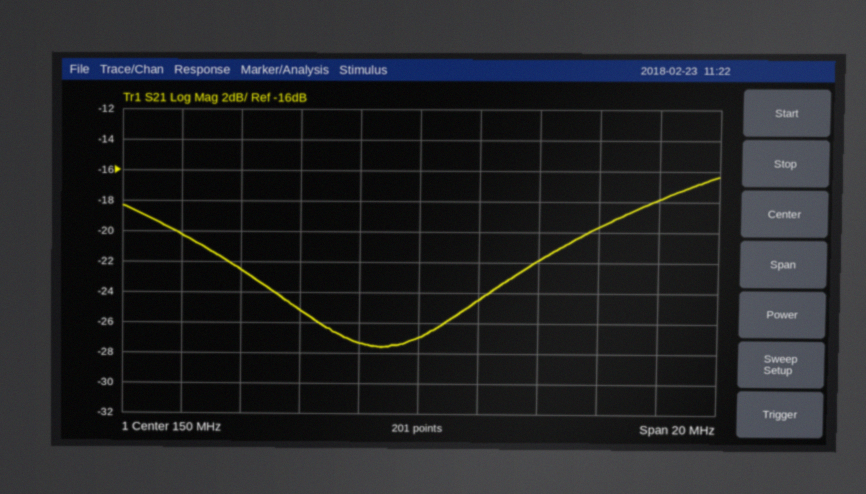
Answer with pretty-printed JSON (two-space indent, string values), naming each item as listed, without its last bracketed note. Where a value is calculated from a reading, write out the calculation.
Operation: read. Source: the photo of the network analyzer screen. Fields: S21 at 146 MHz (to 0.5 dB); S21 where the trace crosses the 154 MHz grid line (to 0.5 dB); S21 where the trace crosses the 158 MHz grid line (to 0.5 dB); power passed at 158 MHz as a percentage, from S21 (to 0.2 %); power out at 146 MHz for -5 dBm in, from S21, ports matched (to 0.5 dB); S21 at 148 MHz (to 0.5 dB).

{
  "S21 at 146 MHz": "-25.0 dB",
  "S21 where the trace crosses the 154 MHz grid line": "-22.0 dB",
  "S21 where the trace crosses the 158 MHz grid line": "-18.0 dB",
  "power passed at 158 MHz as a percentage, from S21": "10^(-18/10) ≈ 1.6 %",
  "power out at 146 MHz for -5 dBm in, from S21, ports matched": "-5 dBm + (-25.0 dB) = -30.0 dBm",
  "S21 at 148 MHz": "-27.5 dB"
}
